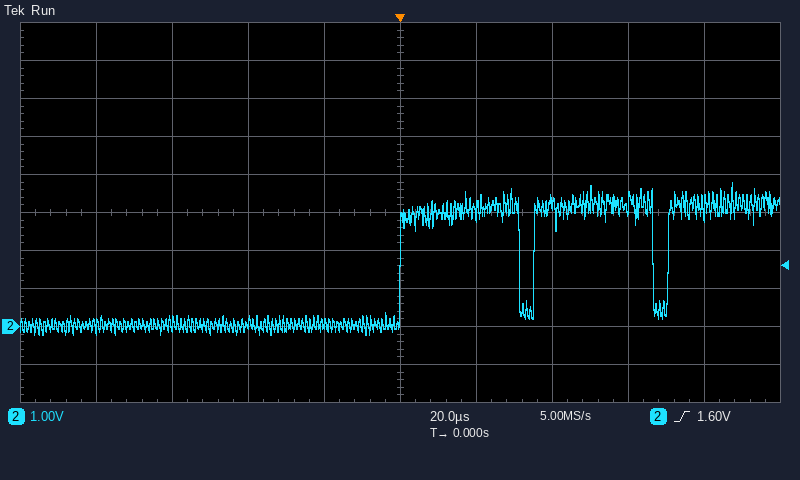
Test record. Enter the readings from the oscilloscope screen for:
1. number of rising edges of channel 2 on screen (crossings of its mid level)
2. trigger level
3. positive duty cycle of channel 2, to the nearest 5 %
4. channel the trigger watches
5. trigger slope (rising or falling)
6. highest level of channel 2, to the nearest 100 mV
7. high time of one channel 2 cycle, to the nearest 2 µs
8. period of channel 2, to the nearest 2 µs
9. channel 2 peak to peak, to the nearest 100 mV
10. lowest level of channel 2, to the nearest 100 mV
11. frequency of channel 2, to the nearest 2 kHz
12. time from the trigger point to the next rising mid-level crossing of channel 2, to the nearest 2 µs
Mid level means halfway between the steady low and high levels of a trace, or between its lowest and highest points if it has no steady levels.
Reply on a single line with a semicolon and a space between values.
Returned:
3; 1.60 V; 90 %; channel 2; rising; 3.8 V; 32 µs; 36 µs; 4.0 V; -200 mV; 28 kHz; 36 µs
